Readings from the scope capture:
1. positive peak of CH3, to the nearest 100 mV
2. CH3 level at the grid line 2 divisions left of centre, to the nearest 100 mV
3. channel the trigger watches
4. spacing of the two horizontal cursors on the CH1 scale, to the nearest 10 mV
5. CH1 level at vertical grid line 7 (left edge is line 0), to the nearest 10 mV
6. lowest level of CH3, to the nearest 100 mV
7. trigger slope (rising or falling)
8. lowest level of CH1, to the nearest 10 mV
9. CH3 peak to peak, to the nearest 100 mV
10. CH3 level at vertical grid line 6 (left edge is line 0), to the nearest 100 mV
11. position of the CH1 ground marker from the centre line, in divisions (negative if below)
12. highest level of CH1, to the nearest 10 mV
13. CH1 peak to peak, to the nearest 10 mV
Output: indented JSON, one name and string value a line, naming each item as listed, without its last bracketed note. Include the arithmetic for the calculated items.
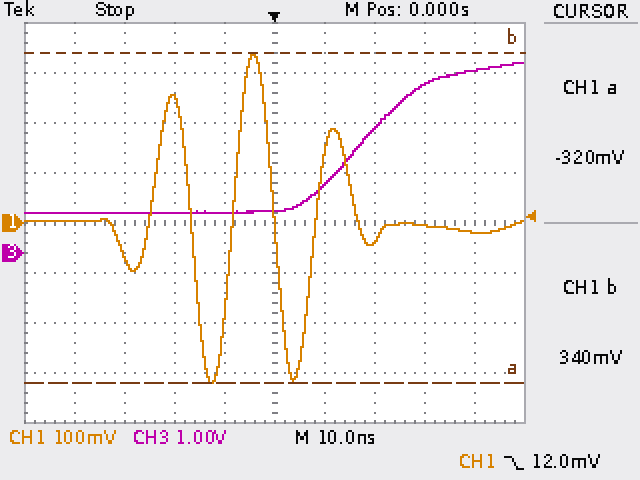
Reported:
{
  "positive peak of CH3, to the nearest 100 mV": "3.8 V",
  "CH3 level at the grid line 2 divisions left of centre, to the nearest 100 mV": "800 mV",
  "channel the trigger watches": "CH1",
  "spacing of the two horizontal cursors on the CH1 scale, to the nearest 10 mV": "660 mV",
  "CH1 level at vertical grid line 7 (left edge is line 0), to the nearest 10 mV": "-40 mV",
  "lowest level of CH3, to the nearest 100 mV": "800 mV",
  "trigger slope": "falling",
  "lowest level of CH1, to the nearest 10 mV": "-320 mV",
  "CH3 peak to peak, to the nearest 100 mV": "3.8 V − (800 mV) = 3.0 V",
  "CH3 level at vertical grid line 6 (left edge is line 0), to the nearest 100 mV": "1.4 V",
  "position of the CH1 ground marker from the centre line, in divisions": "0.0 div",
  "highest level of CH1, to the nearest 10 mV": "340 mV",
  "CH1 peak to peak, to the nearest 10 mV": "340 mV − (-320 mV) = 660 mV"
}
